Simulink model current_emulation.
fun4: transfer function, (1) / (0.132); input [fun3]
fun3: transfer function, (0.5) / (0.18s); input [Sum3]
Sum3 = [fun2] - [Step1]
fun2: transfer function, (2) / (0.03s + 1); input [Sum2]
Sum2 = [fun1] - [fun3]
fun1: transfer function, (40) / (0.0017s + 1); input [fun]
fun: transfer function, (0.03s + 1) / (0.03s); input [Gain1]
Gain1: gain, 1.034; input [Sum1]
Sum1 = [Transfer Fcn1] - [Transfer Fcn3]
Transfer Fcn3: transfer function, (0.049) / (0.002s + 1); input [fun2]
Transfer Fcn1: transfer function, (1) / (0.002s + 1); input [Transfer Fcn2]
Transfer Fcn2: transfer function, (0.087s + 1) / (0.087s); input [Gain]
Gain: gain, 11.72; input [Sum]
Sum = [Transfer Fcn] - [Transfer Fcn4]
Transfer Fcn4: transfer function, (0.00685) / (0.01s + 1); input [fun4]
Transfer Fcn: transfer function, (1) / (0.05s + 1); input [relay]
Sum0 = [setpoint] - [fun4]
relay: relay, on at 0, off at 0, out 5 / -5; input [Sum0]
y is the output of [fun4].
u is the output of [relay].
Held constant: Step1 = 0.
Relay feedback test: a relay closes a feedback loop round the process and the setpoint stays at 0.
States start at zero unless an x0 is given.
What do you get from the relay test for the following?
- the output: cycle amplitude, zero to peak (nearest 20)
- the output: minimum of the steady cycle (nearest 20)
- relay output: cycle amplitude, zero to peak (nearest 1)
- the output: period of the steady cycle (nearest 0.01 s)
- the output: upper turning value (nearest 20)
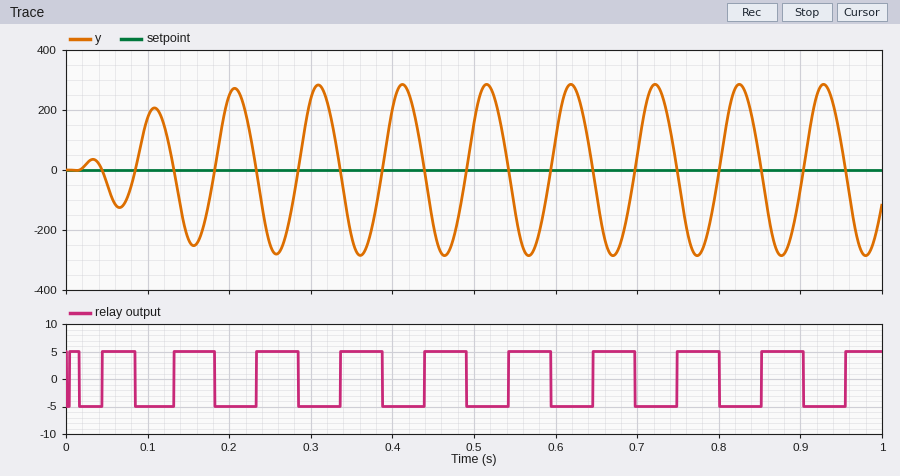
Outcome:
280
-280
5
0.10 s
280
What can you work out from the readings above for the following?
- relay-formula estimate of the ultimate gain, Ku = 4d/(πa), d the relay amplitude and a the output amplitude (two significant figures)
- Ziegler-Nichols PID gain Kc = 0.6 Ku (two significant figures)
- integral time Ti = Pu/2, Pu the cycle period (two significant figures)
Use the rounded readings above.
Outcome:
0.023
0.014
0.050 s
